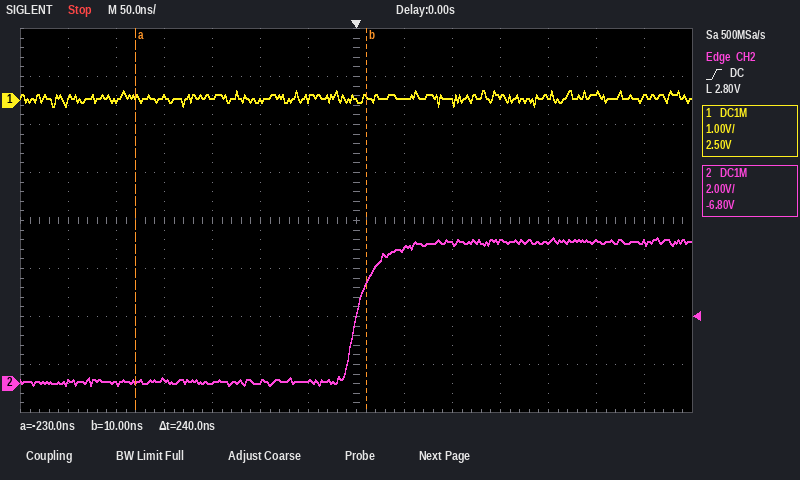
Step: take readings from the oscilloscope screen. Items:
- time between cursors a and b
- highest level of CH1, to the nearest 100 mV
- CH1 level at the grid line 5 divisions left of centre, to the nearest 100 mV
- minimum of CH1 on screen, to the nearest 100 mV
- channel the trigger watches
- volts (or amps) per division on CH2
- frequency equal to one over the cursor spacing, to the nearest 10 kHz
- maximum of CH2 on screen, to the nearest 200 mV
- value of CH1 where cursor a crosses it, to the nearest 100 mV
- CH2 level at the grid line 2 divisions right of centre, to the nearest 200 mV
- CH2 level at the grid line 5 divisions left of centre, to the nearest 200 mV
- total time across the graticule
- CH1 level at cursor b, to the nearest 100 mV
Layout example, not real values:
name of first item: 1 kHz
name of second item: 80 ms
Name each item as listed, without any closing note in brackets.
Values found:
time between cursors a and b: 240 ns
highest level of CH1, to the nearest 100 mV: 200 mV
CH1 level at the grid line 5 divisions left of centre, to the nearest 100 mV: 0.0 V
minimum of CH1 on screen, to the nearest 100 mV: -100 mV
channel the trigger watches: CH2
volts (or amps) per division on CH2: 2 V
frequency equal to one over the cursor spacing, to the nearest 10 kHz: 4.17 MHz
maximum of CH2 on screen, to the nearest 200 mV: 6.0 V
value of CH1 where cursor a crosses it, to the nearest 100 mV: 100 mV
CH2 level at the grid line 2 divisions right of centre, to the nearest 200 mV: 5.8 V
CH2 level at the grid line 5 divisions left of centre, to the nearest 200 mV: 0.0 V
total time across the graticule: 700 ns
CH1 level at cursor b, to the nearest 100 mV: 100 mV
